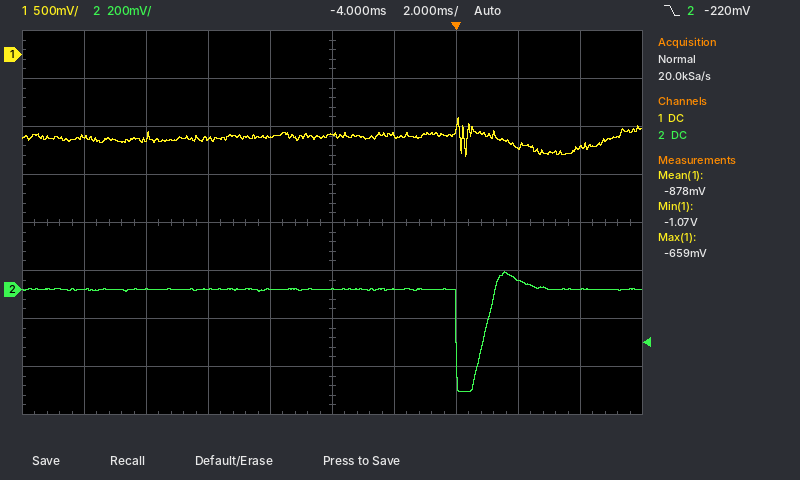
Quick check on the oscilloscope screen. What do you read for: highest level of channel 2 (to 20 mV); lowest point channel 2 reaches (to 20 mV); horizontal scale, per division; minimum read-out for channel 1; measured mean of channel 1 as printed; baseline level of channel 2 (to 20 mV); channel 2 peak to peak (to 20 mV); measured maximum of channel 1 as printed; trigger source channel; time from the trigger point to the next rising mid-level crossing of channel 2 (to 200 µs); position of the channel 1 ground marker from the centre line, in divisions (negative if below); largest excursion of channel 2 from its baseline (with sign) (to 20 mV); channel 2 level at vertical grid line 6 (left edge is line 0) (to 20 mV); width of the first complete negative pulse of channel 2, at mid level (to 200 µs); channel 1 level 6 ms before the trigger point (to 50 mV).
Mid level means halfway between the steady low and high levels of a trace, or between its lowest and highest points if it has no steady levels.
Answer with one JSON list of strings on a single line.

["80 mV", "-420 mV", "2 ms", "-1.07 V", "-878 mV", "0 mV", "500 mV", "-659 mV", "channel 2", "1.0 ms", "+3.5 div", "-420 mV", "0 mV", "1.0 ms", "-850 mV"]
